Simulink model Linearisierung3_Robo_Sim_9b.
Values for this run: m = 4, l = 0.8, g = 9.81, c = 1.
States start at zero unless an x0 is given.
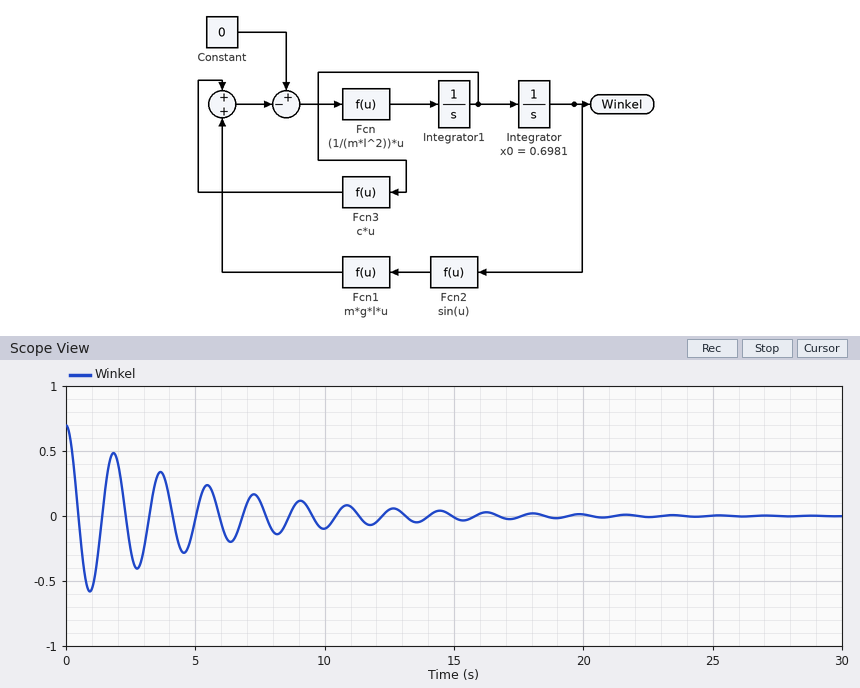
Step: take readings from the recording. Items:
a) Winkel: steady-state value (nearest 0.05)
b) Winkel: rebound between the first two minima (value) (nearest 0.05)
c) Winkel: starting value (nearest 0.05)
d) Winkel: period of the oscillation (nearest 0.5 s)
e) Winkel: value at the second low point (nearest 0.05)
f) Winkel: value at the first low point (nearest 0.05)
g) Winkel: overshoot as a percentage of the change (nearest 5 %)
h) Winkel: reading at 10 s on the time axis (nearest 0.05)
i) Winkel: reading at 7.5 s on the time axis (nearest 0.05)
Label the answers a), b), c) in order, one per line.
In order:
a) 0.00
b) 0.50
c) 0.70
d) 2.0 s
e) -0.40
f) -0.60
g) 85 %
h) -0.10
i) 0.10
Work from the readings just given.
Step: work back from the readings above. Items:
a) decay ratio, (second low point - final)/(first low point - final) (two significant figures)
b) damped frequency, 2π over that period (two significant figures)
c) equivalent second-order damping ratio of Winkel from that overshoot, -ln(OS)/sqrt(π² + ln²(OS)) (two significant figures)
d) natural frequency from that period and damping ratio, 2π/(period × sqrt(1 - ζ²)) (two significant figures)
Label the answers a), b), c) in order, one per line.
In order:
a) 0.67
b) 3.1 rad/s
c) 0.052
d) 3.1 rad/s
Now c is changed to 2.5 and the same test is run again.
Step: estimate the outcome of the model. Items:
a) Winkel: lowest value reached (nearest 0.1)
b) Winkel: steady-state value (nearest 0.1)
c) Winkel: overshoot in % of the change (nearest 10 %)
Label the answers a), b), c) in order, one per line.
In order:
a) -0.4
b) 0.0
c) 60 %
